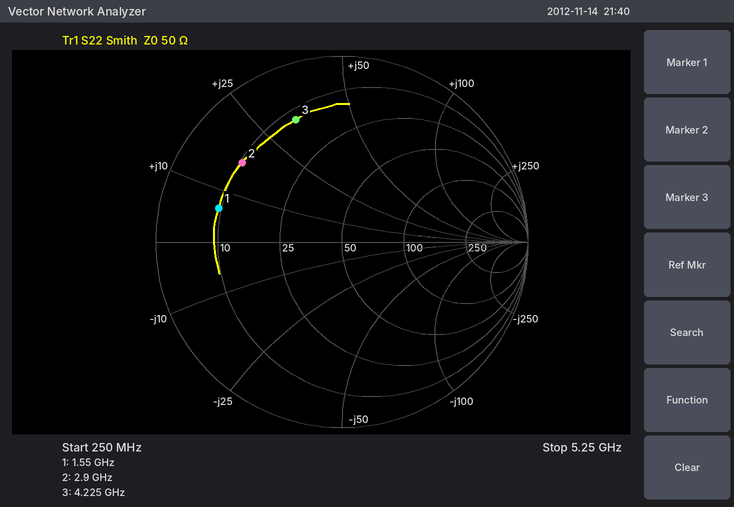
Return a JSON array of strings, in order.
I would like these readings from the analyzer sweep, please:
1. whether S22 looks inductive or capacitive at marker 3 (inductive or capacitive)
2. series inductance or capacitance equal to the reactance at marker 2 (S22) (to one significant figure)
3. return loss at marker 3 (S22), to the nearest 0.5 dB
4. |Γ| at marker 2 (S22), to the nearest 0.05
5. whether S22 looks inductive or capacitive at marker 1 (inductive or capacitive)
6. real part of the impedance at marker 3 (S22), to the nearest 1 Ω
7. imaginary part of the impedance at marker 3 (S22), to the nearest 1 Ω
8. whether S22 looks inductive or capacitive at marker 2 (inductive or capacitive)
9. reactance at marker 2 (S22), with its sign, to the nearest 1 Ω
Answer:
["inductive", "900 pH", "3.0 dB", "0.70", "inductive", "13 Ω", "+33 Ω", "inductive", "+17 Ω"]
